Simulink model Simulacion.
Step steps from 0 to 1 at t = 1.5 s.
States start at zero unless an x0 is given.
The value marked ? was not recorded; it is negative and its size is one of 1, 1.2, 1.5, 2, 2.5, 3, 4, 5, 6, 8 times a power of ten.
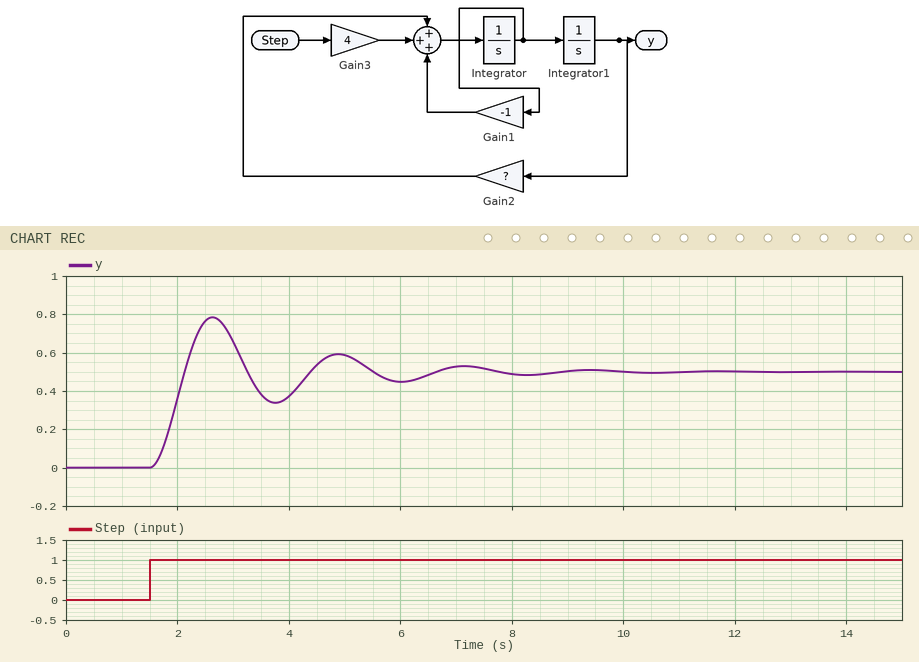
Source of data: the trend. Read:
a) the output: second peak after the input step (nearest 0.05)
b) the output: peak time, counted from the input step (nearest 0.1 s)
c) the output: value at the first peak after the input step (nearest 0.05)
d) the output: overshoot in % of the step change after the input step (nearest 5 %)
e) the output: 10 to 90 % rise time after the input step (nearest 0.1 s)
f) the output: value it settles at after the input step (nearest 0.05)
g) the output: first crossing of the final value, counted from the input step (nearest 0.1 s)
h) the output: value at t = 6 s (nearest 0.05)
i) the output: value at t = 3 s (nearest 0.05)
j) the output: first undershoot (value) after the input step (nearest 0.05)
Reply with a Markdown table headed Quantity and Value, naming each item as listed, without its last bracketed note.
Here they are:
| Quantity | Value |
|---|---|
| the output: second peak after the input step | 0.60 |
| the output: peak time, counted from the input step | 1.1 s |
| the output: value at the first peak after the input step | 0.80 |
| the output: overshoot in % of the step change after the input step | 55 % |
| the output: 10 to 90 % rise time after the input step | 0.4 s |
| the output: value it settles at after the input step | 0.50 |
| the output: first crossing of the final value, counted from the input step | 0.6 s |
| the output: value at t = 6 s | 0.45 |
| the output: value at t = 3 s | 0.65 |
| the output: first undershoot (value) after the input step | 0.35 |
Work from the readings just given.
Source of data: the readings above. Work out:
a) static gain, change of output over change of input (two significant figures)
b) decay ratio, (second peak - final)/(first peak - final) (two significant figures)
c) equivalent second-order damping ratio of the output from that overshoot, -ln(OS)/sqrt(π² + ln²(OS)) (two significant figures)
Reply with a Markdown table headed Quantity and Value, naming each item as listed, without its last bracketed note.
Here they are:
| Quantity | Value |
|---|---|
| static gain, change of output over change of input | 0.50 |
| decay ratio, (second peak - final)/(first peak - final) | 0.33 |
| equivalent second-order damping ratio of the output from that overshoot, -ln(OS)/sqrt(π² + ln²(OS)) | 0.19 |
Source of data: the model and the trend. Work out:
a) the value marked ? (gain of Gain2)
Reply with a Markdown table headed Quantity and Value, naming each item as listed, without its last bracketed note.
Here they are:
| Quantity | Value |
|---|---|
| the value marked ? | -8 |
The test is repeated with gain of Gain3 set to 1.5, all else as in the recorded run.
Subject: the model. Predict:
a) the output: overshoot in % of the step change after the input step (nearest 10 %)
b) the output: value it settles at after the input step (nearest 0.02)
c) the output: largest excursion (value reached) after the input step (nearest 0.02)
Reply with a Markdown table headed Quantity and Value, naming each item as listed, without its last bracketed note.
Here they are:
| Quantity | Value |
|---|---|
| the output: overshoot in % of the step change after the input step | 60 % |
| the output: value it settles at after the input step | 0.18 |
| the output: largest excursion (value reached) after the input step | 0.30 |
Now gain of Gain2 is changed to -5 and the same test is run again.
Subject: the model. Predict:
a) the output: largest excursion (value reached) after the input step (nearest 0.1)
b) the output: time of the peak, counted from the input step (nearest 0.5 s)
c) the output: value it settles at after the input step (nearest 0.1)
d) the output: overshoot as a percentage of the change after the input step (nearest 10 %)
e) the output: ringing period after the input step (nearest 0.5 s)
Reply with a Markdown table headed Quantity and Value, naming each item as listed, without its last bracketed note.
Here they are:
| Quantity | Value |
|---|---|
| the output: largest excursion (value reached) after the input step | 1.2 |
| the output: time of the peak, counted from the input step | 1.5 s |
| the output: value it settles at after the input step | 0.8 |
| the output: overshoot as a percentage of the change after the input step | 50 % |
| the output: ringing period after the input step | 3.0 s |
